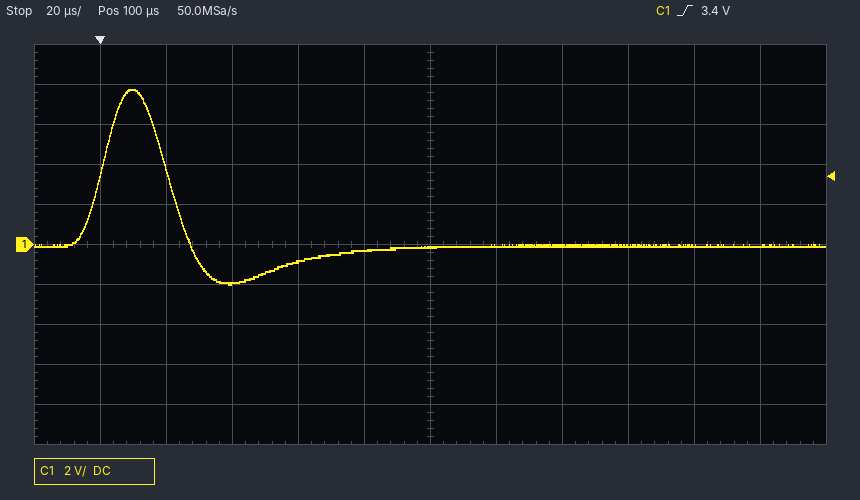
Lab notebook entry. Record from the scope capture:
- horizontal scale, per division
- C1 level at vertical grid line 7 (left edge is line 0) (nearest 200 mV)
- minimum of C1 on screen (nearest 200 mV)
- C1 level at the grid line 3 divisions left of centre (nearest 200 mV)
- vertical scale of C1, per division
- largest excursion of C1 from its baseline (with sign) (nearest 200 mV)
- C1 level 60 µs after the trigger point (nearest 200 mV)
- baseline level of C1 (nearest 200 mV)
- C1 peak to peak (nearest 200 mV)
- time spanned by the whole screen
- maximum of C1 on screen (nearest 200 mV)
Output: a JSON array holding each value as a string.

["20 µs", "0.0 V", "-2.0 V", "-2.0 V", "2 V", "+7.8 V", "-800 mV", "0.0 V", "9.8 V", "240 µs", "7.8 V"]
